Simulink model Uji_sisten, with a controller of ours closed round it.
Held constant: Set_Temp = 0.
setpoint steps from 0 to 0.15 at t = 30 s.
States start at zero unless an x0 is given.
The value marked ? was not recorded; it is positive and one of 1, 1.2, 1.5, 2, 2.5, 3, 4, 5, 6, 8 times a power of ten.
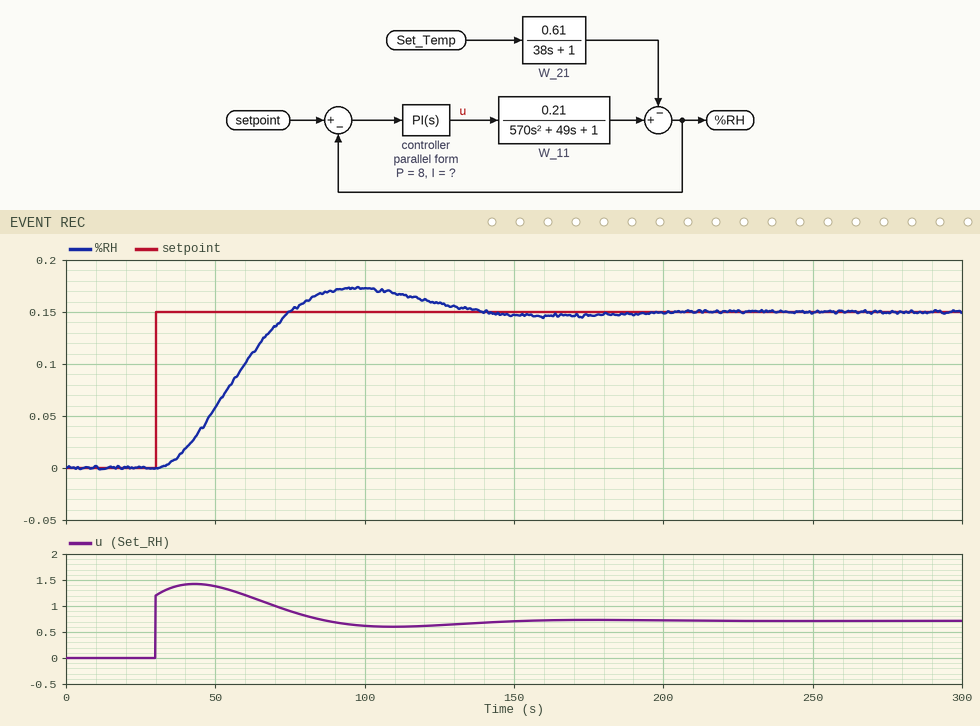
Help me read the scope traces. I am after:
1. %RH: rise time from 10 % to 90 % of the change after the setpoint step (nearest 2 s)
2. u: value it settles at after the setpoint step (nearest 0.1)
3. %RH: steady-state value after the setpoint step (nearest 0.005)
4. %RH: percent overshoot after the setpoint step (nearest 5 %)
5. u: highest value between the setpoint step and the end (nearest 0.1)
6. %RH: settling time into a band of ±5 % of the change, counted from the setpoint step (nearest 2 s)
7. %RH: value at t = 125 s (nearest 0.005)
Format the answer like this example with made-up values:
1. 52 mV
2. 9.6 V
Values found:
1. 30 s
2. 0.7
3. 0.150
4. 15 %
5. 1.4
6. 96 s
7. 0.160
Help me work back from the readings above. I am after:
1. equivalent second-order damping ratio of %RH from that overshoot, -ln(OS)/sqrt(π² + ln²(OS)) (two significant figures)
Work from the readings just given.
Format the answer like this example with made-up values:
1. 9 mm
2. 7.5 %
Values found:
1. 0.52
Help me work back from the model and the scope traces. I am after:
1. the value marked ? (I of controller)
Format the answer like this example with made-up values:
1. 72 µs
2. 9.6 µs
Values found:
1. 0.25
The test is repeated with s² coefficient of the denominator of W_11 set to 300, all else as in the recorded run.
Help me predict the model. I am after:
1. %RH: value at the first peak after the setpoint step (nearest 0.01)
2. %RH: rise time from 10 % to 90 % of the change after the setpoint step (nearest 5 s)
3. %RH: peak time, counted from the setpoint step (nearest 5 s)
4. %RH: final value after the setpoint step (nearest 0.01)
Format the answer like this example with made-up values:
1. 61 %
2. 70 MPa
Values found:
1. 0.16
2. 35 s
3. 75 s
4. 0.15
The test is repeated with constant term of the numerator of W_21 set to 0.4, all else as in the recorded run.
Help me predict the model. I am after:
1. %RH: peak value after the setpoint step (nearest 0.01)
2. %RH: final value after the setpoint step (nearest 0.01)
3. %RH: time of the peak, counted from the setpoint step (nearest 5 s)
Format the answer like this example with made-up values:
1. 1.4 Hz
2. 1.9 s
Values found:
1. 0.17
2. 0.15
3. 65 s
